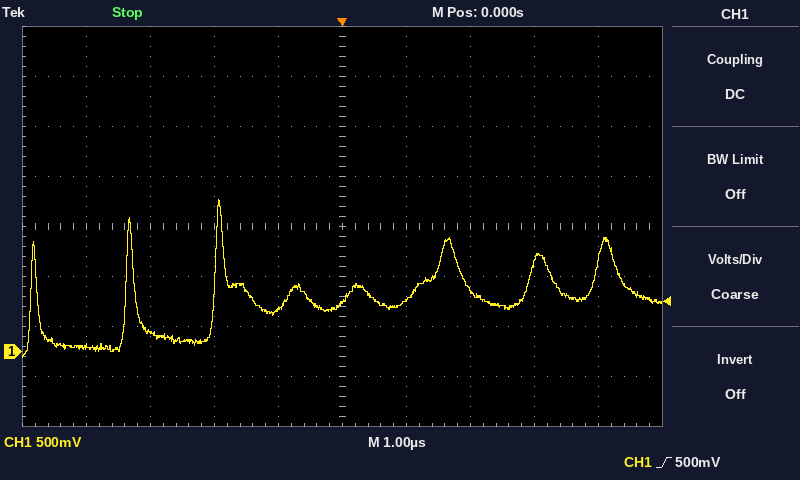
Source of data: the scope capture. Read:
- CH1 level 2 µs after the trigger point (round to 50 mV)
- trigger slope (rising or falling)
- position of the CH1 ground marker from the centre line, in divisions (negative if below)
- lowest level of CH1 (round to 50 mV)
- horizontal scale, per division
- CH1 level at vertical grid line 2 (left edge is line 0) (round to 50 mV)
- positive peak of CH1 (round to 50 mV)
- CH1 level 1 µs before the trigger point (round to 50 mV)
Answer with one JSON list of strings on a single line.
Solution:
["600 mV", "rising", "-2.5 div", "-50 mV", "1 µs", "200 mV", "1.50 V", "400 mV"]
